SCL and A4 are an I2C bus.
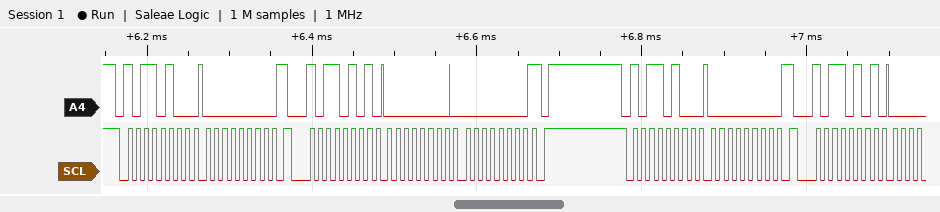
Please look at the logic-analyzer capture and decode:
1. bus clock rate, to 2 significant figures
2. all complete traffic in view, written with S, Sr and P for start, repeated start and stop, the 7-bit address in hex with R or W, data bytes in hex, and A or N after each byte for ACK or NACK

100 kHz
S 5AW A 00 A Sr 5AR A 00 A 00 N P S 5AW A 00 A Sr 5AR A
